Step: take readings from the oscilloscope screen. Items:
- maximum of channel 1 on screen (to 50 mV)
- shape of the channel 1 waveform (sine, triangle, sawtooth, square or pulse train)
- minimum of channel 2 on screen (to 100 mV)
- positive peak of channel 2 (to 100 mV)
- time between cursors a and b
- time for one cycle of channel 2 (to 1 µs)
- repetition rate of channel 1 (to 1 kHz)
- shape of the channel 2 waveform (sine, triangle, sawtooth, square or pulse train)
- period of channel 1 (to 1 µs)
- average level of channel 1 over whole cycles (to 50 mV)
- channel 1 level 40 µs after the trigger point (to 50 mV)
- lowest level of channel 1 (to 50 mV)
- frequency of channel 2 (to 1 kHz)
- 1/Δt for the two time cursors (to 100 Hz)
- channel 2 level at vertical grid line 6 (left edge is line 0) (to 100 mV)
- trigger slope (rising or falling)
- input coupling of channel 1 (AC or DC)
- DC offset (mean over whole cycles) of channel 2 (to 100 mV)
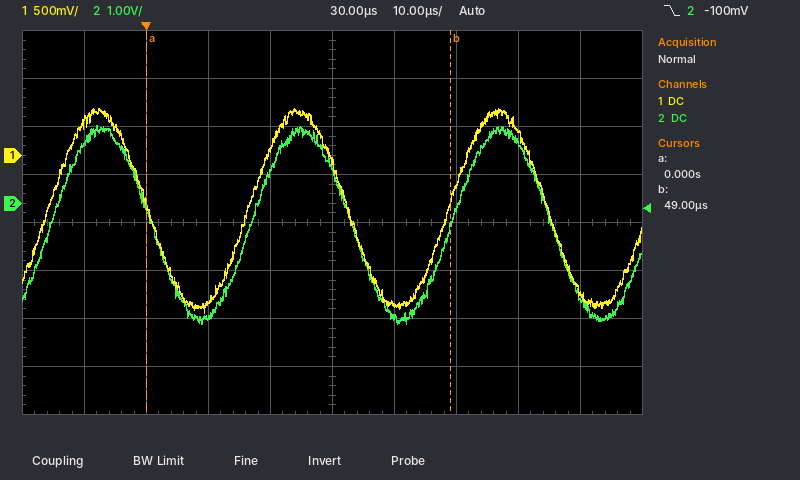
500 mV
sine
-2.5 V
1.6 V
49 µs
32 µs
31 kHz
sine
32 µs
-550 mV
-1.55 V
-1.65 V
31 kHz
20.4 kHz
-2.4 V
falling
DC
-400 mV
